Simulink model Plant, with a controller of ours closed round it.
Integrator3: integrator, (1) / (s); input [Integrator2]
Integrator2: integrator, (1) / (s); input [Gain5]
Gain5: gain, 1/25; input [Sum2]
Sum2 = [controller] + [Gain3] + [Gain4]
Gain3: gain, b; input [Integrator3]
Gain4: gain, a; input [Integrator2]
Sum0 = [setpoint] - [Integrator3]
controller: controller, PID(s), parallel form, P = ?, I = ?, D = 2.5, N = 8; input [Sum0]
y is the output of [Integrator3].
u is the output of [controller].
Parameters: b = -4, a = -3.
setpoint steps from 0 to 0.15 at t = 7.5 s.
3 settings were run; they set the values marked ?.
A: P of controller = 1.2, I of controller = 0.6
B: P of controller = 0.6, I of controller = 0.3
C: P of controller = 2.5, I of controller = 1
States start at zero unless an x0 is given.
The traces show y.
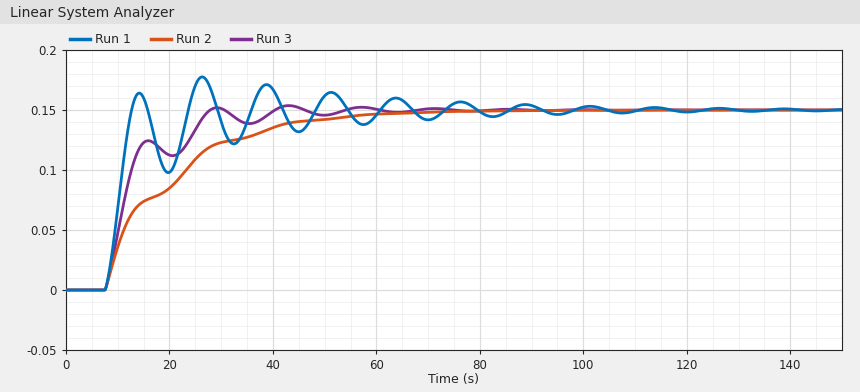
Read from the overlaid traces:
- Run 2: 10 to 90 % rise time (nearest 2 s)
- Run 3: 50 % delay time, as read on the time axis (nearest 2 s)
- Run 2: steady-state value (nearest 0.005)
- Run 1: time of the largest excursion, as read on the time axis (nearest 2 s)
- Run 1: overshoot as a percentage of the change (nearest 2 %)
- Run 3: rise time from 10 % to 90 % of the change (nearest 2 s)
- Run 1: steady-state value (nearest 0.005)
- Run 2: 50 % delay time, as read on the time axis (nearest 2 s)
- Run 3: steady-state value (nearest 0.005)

32 s
12 s
0.150
26 s
18 %
16 s
0.150
16 s
0.150
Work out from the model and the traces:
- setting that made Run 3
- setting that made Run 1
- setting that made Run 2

A
C
B
